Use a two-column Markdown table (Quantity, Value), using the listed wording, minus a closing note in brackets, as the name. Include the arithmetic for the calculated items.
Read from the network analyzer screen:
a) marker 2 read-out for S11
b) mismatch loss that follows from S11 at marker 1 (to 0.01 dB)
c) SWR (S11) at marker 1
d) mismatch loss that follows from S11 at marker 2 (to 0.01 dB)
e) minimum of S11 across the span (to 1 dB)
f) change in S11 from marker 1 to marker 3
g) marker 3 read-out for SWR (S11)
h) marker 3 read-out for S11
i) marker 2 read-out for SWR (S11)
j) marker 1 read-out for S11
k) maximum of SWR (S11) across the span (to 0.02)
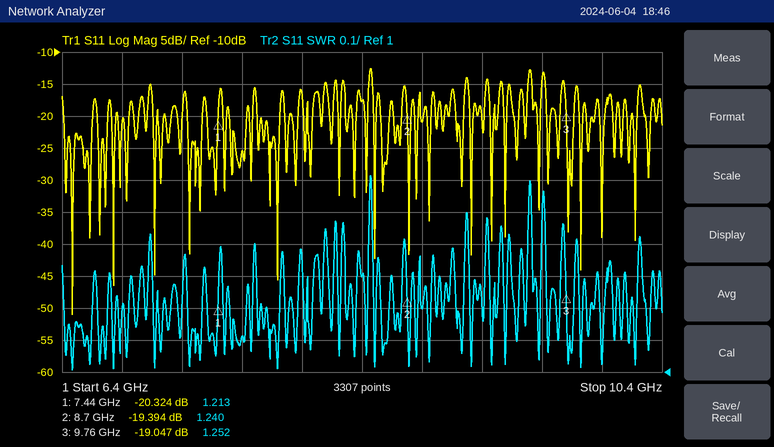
| Quantity | Value |
|---|---|
| marker 2 read-out for S11 | -19.394 dB |
| mismatch loss that follows from S11 at marker 1 | −10 log10(1 − 10^(-20.324/10)) ≈ 0.04 dB |
| SWR (S11) at marker 1 | 1.213 |
| mismatch loss that follows from S11 at marker 2 | −10 log10(1 − 10^(-19.394/10)) ≈ 0.05 dB |
| minimum of S11 across the span | -51 dB |
| change in S11 from marker 1 to marker 3 | -19.047 − (-20.324) = 1.277 dB |
| marker 3 read-out for SWR | 1.252 |
| marker 3 read-out for S11 | -19.047 dB |
| marker 2 read-out for SWR | 1.240 |
| marker 1 read-out for S11 | -20.324 dB |
| maximum of SWR (S11) across the span | 1.62 |
